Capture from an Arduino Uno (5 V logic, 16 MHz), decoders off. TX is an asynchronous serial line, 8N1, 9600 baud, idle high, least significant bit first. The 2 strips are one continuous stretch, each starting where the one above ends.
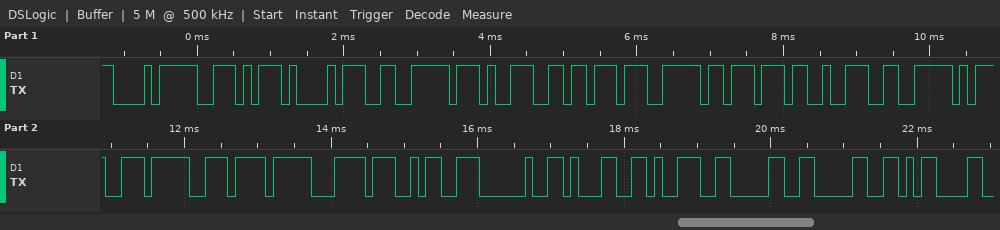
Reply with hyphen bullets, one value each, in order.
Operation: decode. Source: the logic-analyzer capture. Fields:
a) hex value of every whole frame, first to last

- 0xE8 0xAE 0xA1 0xE6 0x97 0xB6 0xE7 0xBB 0x93 0xE6 0x9D 0x9F 0xEF 0xBC 0x9A 0x20 0x31 0x39 0x30 0x30 0x0D
